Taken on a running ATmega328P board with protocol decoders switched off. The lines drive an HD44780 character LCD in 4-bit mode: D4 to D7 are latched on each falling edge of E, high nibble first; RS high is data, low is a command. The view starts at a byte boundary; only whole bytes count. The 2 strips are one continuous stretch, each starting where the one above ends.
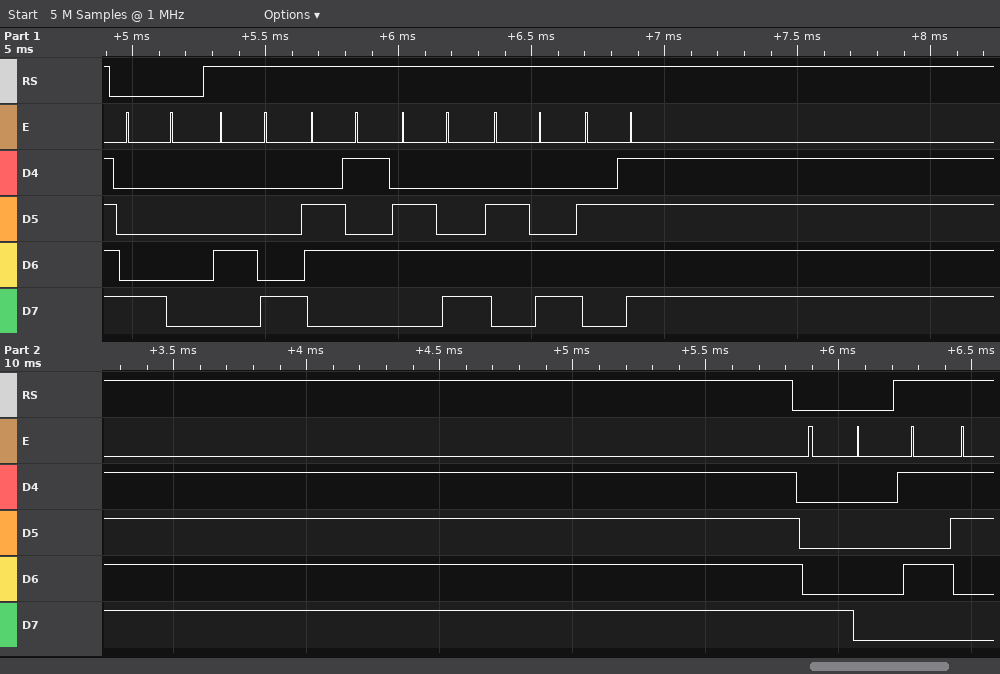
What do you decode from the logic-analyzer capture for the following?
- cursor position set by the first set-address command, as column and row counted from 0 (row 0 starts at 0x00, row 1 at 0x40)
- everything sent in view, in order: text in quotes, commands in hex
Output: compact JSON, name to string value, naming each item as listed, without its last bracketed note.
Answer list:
{"cursor position set by the first set-address command, as column and row counted from 0": "column 0, row 0", "everything sent in view, in order: text in quotes, commands in hex": "0x80 \"Hello\" 0x80 \"S\""}
